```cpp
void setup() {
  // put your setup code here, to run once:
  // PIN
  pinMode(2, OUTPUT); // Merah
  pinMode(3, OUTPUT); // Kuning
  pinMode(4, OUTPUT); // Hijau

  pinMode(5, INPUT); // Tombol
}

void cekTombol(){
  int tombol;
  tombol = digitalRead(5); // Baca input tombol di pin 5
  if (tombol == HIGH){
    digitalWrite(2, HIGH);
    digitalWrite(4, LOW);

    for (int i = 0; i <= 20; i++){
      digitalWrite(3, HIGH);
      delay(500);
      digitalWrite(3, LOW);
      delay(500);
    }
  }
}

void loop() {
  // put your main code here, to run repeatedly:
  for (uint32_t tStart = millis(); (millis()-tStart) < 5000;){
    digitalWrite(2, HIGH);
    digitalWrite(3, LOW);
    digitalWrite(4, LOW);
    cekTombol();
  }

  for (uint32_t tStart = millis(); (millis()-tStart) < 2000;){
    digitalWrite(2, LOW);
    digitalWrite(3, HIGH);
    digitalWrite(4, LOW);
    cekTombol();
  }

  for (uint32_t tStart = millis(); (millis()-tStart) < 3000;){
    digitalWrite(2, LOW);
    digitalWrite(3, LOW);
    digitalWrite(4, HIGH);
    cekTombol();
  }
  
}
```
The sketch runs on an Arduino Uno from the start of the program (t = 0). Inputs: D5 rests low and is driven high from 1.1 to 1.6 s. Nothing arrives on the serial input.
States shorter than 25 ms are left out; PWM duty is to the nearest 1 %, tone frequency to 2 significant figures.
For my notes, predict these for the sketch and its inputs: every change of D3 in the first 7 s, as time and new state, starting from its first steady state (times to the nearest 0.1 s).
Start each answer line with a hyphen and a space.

- 0 s low; 1.1 s high; 1.6 s low; 2.1 s high; 2.6 s low; 3.1 s high; 3.6 s low; 4.1 s high; 4.6 s low; 5.1 s high; 5.6 s low; 6.1 s high; 6.6 s low
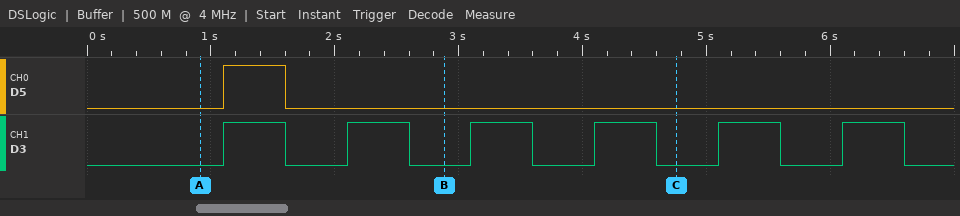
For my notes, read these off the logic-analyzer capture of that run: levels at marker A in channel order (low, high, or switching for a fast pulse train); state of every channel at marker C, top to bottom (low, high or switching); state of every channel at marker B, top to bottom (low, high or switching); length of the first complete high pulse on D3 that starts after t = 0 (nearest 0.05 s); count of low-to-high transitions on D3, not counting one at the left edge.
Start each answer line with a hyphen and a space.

- D5 low, D3 low
- D5 low, D3 low
- D5 low, D3 low
- 0.50 s
- 6
